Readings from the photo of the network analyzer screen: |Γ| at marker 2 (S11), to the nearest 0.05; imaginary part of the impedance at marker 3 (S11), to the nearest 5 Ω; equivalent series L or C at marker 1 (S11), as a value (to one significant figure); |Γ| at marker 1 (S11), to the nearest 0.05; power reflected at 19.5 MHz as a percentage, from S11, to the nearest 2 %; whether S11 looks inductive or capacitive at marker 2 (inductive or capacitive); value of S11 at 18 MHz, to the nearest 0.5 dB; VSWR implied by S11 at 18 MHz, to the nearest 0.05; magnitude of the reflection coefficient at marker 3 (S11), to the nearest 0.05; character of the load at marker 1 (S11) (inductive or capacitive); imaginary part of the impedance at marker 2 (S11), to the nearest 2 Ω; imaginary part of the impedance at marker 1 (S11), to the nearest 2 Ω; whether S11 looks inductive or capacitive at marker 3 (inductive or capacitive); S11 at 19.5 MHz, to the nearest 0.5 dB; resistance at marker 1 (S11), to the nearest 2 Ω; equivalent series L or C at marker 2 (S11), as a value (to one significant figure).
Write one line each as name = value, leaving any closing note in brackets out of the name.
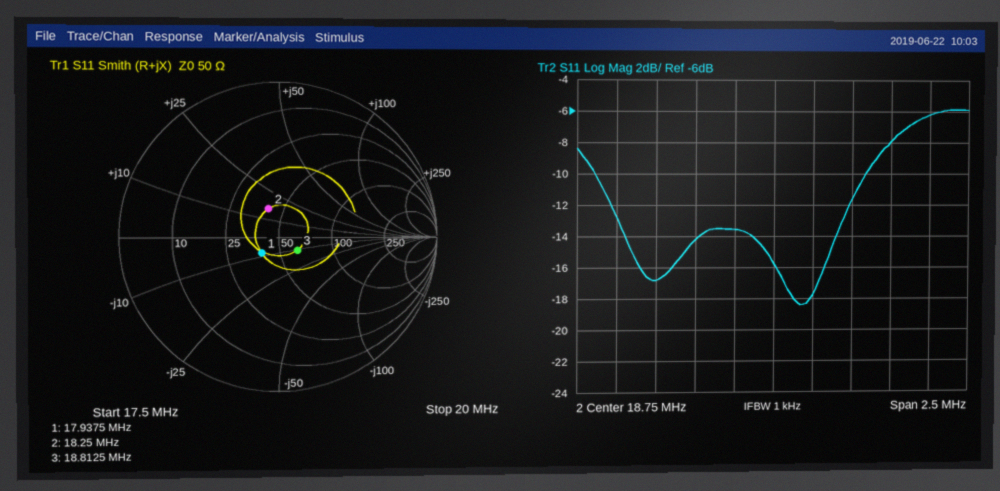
|Γ| at marker 2 (S11), to the nearest 0.05 = 0.20
imaginary part of the impedance at marker 3 (S11), to the nearest 5 Ω = -10 Ω
equivalent series L or C at marker 1 (S11), as a value = 1 nF
|Γ| at marker 1 (S11), to the nearest 0.05 = 0.15
power reflected at 19.5 MHz as a percentage, from S11, to the nearest 2 % = 16 %
whether S11 looks inductive or capacitive at marker 2 = inductive
value of S11 at 18 MHz, to the nearest 0.5 dB = -17.0 dB
VSWR implied by S11 at 18 MHz, to the nearest 0.05 = 1.35
magnitude of the reflection coefficient at marker 3 (S11), to the nearest 0.05 = 0.15
character of the load at marker 1 (S11) = capacitive
imaginary part of the impedance at marker 2 (S11), to the nearest 2 Ω = +16 Ω
imaginary part of the impedance at marker 1 (S11), to the nearest 2 Ω = -8 Ω
whether S11 looks inductive or capacitive at marker 3 = capacitive
S11 at 19.5 MHz, to the nearest 0.5 dB = -8.0 dB
resistance at marker 1 (S11), to the nearest 2 Ω = 40 Ω
equivalent series L or C at marker 2 (S11), as a value = 100 nH
